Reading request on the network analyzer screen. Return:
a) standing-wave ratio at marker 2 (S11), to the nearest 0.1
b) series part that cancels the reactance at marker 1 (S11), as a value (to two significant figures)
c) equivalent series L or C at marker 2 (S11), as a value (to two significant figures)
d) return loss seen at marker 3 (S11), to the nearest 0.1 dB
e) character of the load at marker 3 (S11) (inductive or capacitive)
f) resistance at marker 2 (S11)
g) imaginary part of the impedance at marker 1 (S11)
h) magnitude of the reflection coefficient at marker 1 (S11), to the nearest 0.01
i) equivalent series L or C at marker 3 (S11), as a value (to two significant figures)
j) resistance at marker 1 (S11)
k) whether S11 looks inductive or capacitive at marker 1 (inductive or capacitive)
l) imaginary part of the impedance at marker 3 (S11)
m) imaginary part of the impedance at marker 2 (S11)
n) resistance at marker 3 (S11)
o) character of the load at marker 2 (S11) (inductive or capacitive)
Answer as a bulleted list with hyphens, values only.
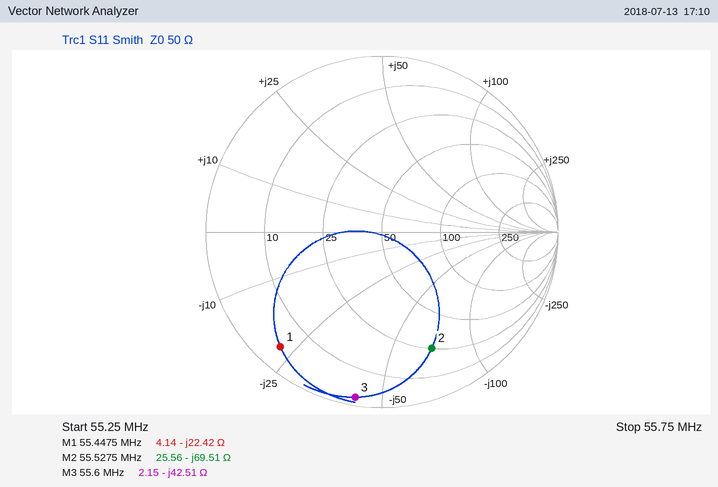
- 6.1
- 64 nH
- 41 pF
- 0.4 dB
- capacitive
- 25.56 Ω
- -22.42 Ω
- 0.87
- 67 pF
- 4.14 Ω
- capacitive
- -42.51 Ω
- -69.51 Ω
- 2.15 Ω
- capacitive
